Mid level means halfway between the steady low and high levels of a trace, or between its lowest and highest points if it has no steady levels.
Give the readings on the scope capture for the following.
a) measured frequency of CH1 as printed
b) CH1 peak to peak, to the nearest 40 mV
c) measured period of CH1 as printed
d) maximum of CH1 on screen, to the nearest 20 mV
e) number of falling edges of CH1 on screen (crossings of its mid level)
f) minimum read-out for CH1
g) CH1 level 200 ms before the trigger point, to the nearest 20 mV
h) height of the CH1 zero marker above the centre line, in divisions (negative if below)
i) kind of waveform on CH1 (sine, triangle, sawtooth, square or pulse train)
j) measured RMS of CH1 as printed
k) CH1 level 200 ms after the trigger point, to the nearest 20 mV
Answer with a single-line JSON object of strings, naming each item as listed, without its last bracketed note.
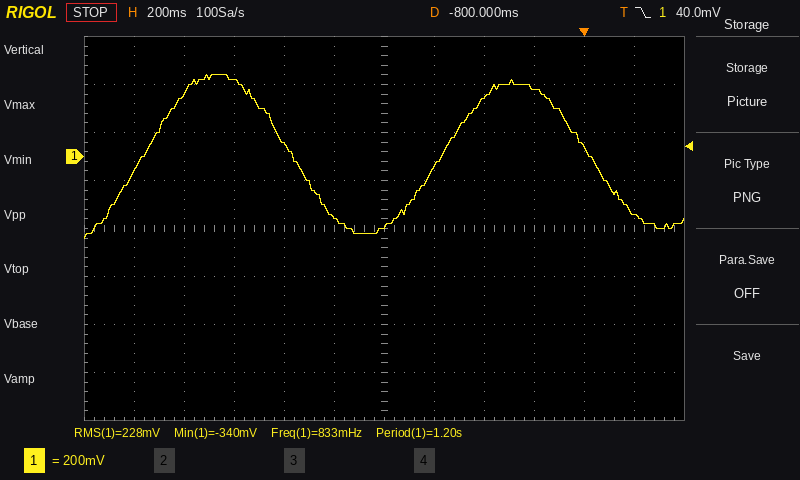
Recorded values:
{"measured frequency of CH1 as printed": "833 mHz", "CH1 peak to peak, to the nearest 40 mV": "680 mV", "measured period of CH1 as printed": "1.20 s", "maximum of CH1 on screen, to the nearest 20 mV": "340 mV", "number of falling edges of CH1 on screen": "2", "minimum read-out for CH1": "-340 mV", "CH1 level 200 ms before the trigger point, to the nearest 20 mV": "280 mV", "height of the CH1 zero marker above the centre line, in divisions": "+1.5 div", "kind of waveform on CH1": "sine", "measured RMS of CH1 as printed": "228 mV", "CH1 level 200 ms after the trigger point, to the nearest 20 mV": "-240 mV"}
